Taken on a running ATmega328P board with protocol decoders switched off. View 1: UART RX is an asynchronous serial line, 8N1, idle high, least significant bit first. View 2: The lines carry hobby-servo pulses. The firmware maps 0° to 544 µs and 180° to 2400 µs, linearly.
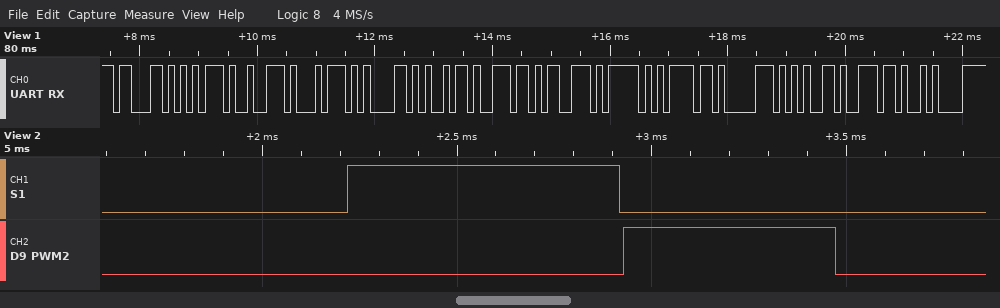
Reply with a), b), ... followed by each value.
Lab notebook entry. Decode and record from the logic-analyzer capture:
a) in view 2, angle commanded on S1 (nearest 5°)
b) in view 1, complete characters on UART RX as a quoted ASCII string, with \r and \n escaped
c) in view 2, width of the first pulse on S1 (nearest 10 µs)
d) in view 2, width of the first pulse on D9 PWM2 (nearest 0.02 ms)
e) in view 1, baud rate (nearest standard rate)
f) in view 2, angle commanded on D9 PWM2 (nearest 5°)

a) 15°
b) "curtains_open\n"
c) 700 µs
d) 0.54 ms
e) 9600 baud
f) 0°
